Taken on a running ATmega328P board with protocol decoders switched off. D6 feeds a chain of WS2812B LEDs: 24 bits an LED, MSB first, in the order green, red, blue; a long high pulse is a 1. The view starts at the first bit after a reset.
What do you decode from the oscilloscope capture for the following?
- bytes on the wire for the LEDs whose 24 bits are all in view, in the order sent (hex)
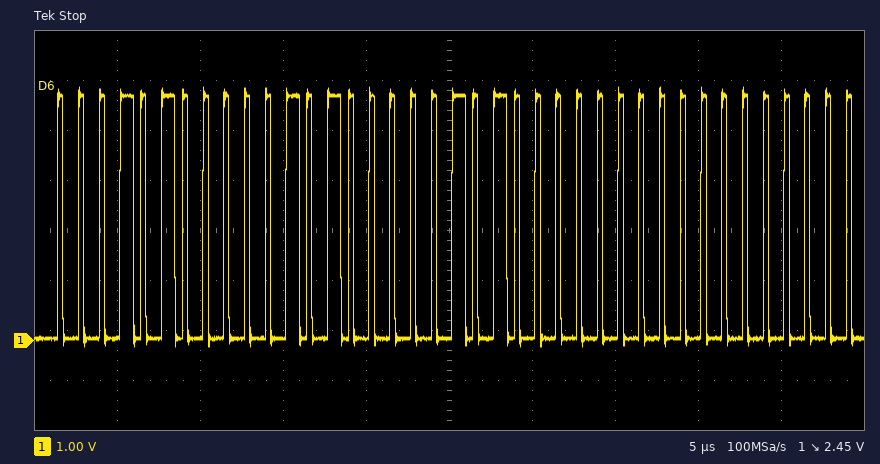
14 14 14
